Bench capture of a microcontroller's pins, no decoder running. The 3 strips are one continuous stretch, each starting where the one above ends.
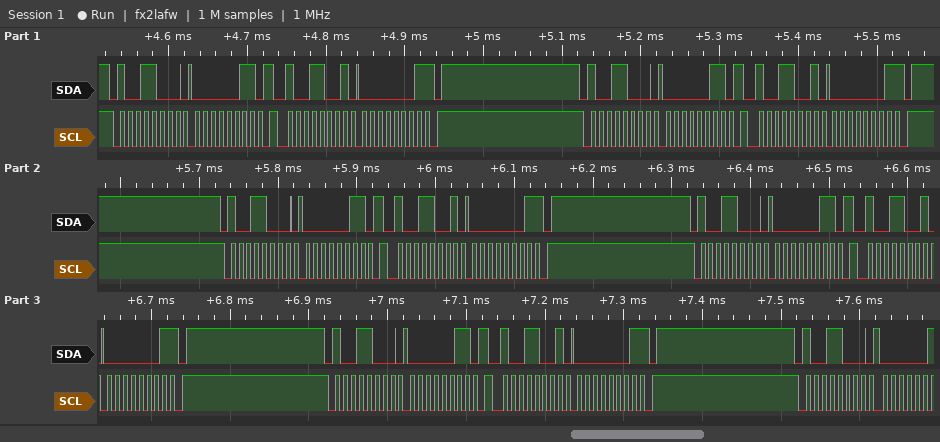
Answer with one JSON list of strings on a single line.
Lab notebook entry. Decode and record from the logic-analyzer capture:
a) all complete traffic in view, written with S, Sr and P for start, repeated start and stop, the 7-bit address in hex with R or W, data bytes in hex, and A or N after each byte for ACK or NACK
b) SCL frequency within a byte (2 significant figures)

["S 4CW A 03 A Sr 4CR A 01 N P S 4CW A 03 A Sr 4CR A 01 N P S 4CW A 03 A Sr 4CR A 01 N P S 4CW A 03 A Sr 4CR A 01 N P S 4CW A 03 A Sr 4CR A 01 N P S 4CW A", "100 kHz"]
